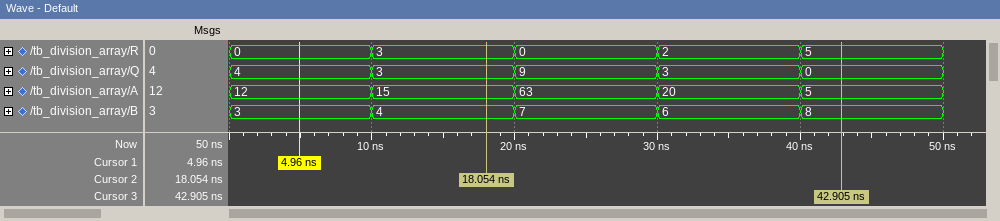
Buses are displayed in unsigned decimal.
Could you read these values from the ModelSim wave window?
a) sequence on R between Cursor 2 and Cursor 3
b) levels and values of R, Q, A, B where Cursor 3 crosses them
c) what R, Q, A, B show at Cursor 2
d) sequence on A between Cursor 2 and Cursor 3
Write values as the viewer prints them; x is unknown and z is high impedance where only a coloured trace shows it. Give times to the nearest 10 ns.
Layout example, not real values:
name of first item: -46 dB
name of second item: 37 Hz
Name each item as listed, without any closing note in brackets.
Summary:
sequence on R between Cursor 2 and Cursor 3: 3, 0, 2, 5
levels and values of R, Q, A, B where Cursor 3 crosses them: R=5, Q=0, A=5, B=8
what R, Q, A, B show at Cursor 2: R=3, Q=3, A=15, B=4
sequence on A between Cursor 2 and Cursor 3: 15, 63, 20, 5
